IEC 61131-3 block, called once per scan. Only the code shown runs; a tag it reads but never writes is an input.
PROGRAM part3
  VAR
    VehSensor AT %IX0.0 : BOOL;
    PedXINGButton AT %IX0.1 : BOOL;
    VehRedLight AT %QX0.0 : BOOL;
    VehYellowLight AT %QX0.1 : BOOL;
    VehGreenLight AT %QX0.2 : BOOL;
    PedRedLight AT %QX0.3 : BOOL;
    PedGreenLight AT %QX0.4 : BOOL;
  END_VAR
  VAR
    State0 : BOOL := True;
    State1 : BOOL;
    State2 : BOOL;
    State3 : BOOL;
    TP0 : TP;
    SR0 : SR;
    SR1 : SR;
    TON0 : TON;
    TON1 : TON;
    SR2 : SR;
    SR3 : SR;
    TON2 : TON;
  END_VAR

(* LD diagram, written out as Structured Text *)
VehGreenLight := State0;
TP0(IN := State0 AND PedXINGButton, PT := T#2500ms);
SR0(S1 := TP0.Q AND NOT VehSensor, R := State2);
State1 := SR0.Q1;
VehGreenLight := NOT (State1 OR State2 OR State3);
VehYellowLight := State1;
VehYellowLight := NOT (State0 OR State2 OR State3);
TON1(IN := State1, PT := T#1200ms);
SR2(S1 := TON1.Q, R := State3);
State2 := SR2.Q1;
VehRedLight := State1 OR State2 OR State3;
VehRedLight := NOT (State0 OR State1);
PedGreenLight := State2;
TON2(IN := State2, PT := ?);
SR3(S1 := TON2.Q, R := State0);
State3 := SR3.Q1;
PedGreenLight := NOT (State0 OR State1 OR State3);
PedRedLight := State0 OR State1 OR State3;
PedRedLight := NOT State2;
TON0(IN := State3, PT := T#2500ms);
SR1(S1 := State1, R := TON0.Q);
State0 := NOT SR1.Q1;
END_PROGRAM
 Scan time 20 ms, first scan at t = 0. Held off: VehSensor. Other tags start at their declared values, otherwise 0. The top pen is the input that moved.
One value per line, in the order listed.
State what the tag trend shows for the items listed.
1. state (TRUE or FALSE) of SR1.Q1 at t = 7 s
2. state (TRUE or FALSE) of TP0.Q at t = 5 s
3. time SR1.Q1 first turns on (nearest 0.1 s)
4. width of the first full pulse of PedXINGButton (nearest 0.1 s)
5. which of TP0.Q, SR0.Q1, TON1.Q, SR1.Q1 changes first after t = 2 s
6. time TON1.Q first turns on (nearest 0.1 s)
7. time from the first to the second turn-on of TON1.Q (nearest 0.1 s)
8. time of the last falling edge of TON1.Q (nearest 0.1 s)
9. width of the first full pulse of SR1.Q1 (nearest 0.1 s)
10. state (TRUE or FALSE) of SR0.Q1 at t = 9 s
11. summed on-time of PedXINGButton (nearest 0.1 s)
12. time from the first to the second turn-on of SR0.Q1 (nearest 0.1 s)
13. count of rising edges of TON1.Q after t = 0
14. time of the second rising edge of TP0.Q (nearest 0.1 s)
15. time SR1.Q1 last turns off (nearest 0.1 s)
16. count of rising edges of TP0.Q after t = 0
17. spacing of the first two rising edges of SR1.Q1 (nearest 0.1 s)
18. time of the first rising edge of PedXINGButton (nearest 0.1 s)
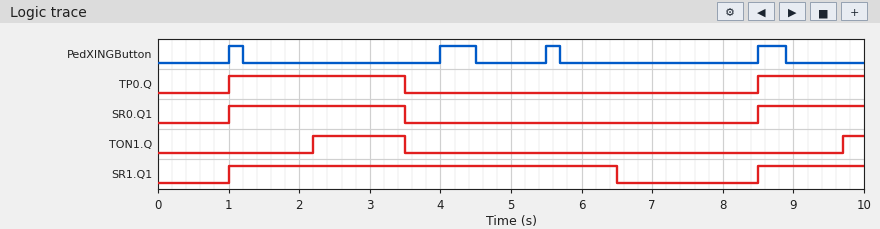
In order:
FALSE
FALSE
1.0 s
0.2 s
TON1.Q
2.2 s
7.5 s
3.5 s
5.5 s
TRUE
1.3 s
7.5 s
2
8.5 s
6.5 s
2
7.5 s
1.0 s
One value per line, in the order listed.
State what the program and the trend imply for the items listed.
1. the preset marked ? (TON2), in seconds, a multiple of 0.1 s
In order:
1.8 s
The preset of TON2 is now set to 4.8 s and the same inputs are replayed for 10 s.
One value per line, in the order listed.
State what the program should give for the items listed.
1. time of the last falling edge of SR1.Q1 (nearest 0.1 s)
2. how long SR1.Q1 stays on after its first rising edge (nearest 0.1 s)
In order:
9.5 s
8.5 s
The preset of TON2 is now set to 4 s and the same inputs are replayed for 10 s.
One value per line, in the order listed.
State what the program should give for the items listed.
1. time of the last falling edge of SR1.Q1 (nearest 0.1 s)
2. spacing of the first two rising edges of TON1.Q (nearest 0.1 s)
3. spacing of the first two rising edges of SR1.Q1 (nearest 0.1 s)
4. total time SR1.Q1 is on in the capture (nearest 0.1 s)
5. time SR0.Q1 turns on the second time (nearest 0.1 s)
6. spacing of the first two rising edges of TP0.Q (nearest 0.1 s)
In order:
8.7 s
7.7 s
7.7 s
9.0 s
8.7 s
7.7 s
